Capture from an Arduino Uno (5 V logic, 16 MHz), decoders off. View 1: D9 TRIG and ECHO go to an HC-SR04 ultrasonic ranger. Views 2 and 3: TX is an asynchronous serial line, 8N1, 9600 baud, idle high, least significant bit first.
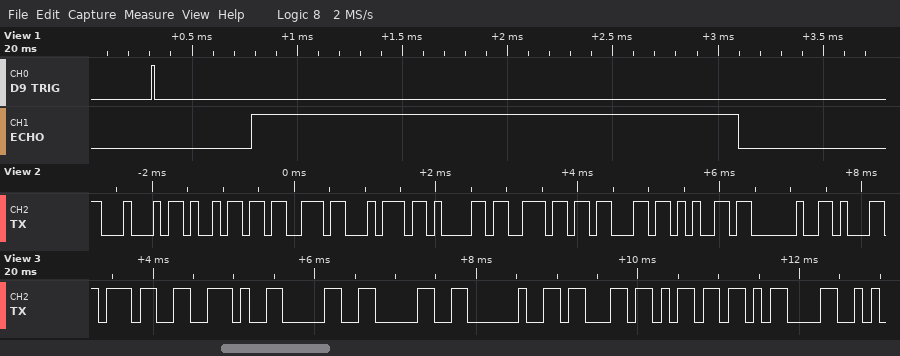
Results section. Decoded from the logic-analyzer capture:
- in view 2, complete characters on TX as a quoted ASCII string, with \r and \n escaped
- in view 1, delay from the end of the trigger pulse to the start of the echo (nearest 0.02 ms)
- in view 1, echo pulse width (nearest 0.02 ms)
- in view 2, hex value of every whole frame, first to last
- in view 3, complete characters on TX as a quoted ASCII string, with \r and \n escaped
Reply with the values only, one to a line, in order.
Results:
"Distance "
0.46 ms
2.32 ms
44 69 73 74 61 6E 63 65 20
"7.00 cm\r"
